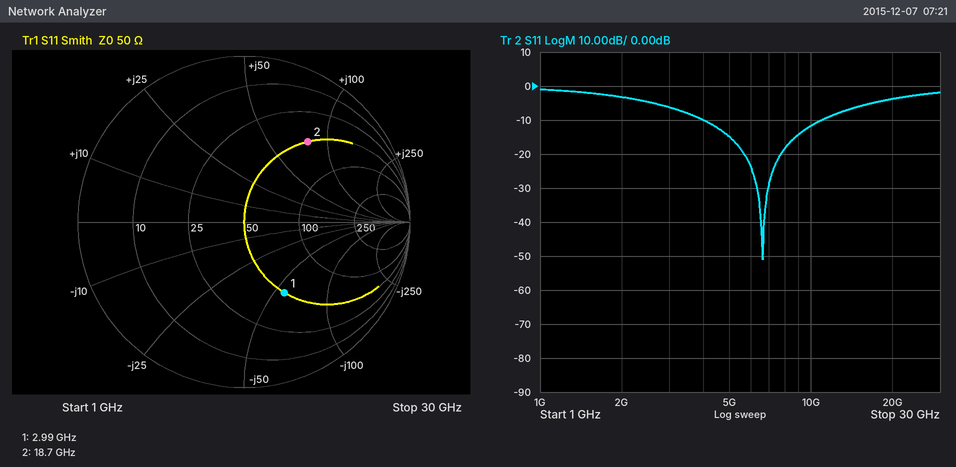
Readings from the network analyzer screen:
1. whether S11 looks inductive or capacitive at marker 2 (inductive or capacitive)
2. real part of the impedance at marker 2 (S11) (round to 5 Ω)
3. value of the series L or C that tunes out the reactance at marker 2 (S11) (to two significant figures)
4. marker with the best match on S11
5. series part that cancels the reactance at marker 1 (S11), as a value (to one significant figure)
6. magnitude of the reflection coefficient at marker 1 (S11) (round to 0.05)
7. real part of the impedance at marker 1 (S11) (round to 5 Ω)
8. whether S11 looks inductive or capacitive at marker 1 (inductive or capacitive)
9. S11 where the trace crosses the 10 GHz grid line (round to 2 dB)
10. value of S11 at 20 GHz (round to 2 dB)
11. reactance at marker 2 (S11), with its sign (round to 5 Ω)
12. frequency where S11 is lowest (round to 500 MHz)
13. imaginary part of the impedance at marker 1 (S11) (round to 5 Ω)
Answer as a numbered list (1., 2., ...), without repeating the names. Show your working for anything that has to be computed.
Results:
1. inductive
2. 50 Ω
3. C = 1/(2π × 18.7 GHz × 80 Ω) ≈ 106 fF, so 110 fF to two significant figures
4. marker 1
5. L = 55 Ω/(2π × 2.99 GHz) ≈ 3 nH
6. 0.50
7. 50 Ω
8. capacitive
9. -12 dB
10. -4 dB
11. +80 Ω
12. 6.5 GHz
13. -55 Ω
